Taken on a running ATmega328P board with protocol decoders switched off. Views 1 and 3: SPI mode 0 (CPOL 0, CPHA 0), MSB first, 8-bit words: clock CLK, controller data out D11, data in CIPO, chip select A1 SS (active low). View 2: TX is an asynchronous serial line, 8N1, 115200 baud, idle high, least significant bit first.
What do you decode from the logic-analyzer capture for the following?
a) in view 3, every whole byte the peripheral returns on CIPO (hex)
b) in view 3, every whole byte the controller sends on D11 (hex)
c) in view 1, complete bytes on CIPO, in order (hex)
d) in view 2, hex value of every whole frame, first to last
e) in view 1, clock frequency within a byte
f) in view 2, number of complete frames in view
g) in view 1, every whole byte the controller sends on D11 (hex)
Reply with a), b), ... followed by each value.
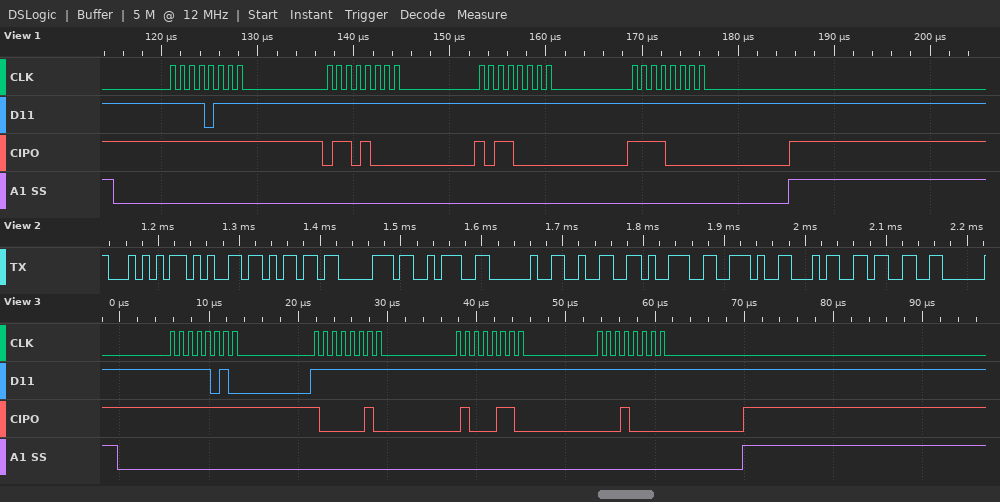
a) FF 82 46 10
b) FA FF FF FF
c) FF 68 B0 F0
d) 0x54 0x65 0x6D 0x70 0x3A 0x20 0x32 0x39 0x2E 0x34 0x33
e) 1 MHz
f) 11
g) F7 FF FF FF
